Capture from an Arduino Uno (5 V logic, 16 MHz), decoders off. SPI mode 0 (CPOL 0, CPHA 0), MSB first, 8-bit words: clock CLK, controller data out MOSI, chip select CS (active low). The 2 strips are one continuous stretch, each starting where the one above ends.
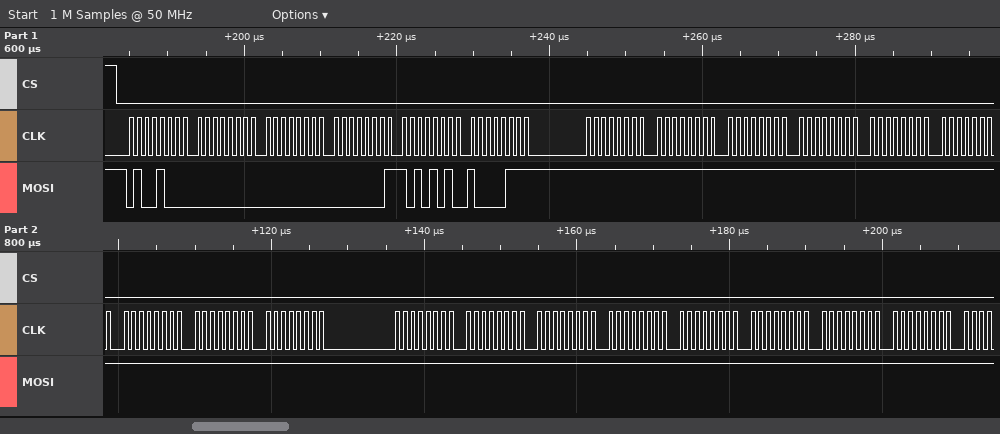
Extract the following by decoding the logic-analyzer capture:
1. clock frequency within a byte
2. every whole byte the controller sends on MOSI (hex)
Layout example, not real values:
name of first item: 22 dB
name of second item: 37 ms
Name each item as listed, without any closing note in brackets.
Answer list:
clock frequency within a byte: 1 MHz
every whole byte the controller sends on MOSI: 48 00 00 01 AA 87 FF FF FF FF FF FF FF FF FF FF FF FF FF FF FF FF FF
